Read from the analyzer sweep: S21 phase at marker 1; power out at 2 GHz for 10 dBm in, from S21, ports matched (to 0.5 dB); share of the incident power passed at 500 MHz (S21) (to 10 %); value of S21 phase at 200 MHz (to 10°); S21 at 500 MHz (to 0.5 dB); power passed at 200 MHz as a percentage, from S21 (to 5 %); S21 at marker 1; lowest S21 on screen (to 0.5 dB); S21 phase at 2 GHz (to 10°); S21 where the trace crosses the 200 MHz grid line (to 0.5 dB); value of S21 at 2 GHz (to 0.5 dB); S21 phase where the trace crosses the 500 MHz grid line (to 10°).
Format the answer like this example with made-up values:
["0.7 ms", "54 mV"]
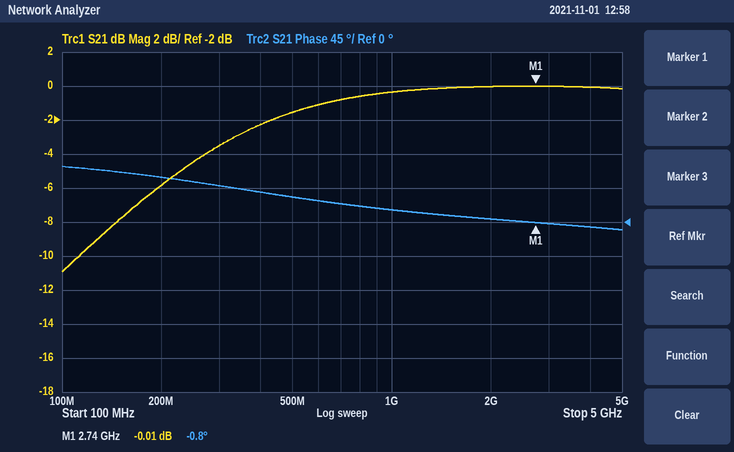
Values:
["-0.8°", "10.0 dBm", "70 %", "60°", "-1.5 dB", "25 %", "-0.01 dB", "-11.0 dB", "0°", "-6.0 dB", "0.0 dB", "30°"]
